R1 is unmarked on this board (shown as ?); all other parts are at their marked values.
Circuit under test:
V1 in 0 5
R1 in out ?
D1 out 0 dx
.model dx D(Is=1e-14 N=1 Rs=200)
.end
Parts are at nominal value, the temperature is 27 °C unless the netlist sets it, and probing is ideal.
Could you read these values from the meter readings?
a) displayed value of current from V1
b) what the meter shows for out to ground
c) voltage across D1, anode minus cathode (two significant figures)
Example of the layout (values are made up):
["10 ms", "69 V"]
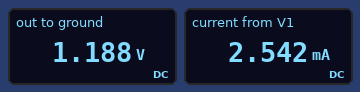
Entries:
["2.542 mA", "1.188 V", "1.2 V"]
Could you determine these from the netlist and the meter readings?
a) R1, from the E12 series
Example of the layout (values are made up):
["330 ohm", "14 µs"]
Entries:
["1.5 kΩ"]
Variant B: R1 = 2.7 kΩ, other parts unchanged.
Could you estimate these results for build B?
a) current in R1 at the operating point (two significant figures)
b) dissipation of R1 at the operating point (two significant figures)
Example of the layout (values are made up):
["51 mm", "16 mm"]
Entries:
["1.5 mA", "6.0 mW"]
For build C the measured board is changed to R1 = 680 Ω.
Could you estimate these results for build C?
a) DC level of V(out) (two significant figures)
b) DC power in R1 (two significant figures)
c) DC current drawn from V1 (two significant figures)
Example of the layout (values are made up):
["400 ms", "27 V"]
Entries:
["1.7 V", "16 mW", "4.9 mA"]
